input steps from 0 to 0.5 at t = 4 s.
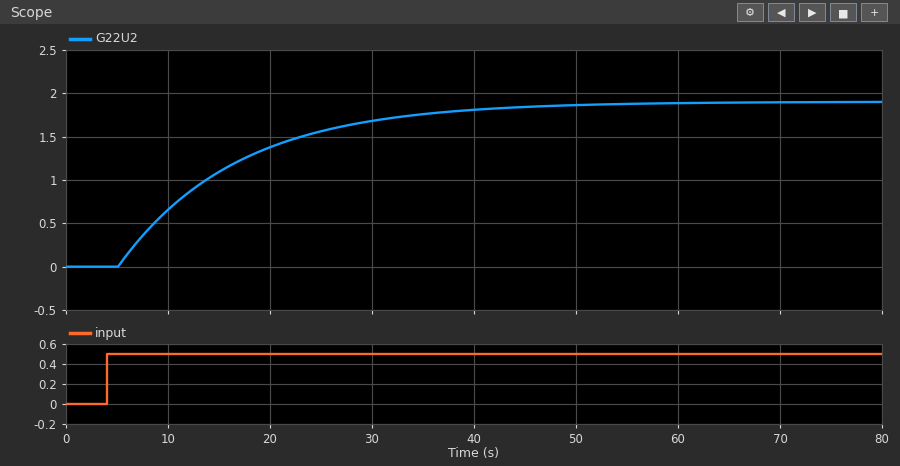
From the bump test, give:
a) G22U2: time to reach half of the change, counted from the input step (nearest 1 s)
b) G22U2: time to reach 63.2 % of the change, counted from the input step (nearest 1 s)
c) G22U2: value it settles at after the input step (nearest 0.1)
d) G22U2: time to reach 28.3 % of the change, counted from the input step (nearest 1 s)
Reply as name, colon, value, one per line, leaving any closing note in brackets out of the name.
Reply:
G22U2: time to reach half of the change, counted from the input step: 9 s
G22U2: time to reach 63.2 % of the change, counted from the input step: 13 s
G22U2: value it settles at after the input step: 1.9
G22U2: time to reach 28.3 % of the change, counted from the input step: 5 s
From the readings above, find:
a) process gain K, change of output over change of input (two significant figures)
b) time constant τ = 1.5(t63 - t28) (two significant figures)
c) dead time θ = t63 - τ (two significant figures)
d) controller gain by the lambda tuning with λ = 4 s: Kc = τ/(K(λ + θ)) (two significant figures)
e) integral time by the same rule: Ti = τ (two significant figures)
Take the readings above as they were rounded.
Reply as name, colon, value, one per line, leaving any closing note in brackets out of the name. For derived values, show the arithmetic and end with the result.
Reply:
process gain K, change of output over change of input: (1.9 - 0) / 0.5 = 3.8
time constant τ = 1.5(t63 - t28): 1.5 × (13 - 5) = 12 s
dead time θ = t63 - τ: 13 - 12 = 1.0 s
controller gain by the lambda tuning with λ = 4 s: Kc = τ/(K(λ + θ)): 12 / (3.8 × (4 + 1)) = 0.63
integral time by the same rule: Ti = τ: 12 s
